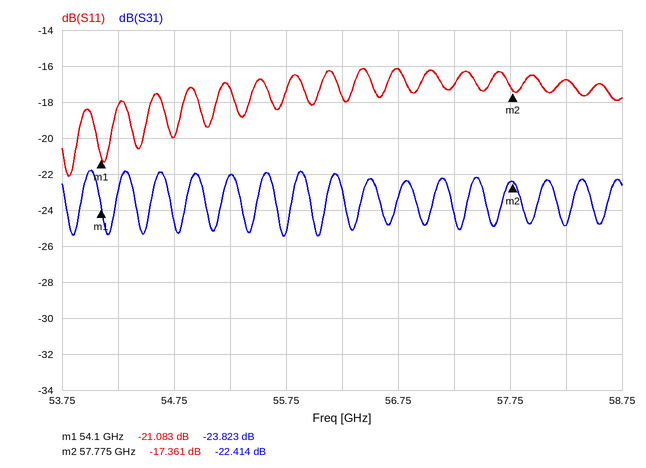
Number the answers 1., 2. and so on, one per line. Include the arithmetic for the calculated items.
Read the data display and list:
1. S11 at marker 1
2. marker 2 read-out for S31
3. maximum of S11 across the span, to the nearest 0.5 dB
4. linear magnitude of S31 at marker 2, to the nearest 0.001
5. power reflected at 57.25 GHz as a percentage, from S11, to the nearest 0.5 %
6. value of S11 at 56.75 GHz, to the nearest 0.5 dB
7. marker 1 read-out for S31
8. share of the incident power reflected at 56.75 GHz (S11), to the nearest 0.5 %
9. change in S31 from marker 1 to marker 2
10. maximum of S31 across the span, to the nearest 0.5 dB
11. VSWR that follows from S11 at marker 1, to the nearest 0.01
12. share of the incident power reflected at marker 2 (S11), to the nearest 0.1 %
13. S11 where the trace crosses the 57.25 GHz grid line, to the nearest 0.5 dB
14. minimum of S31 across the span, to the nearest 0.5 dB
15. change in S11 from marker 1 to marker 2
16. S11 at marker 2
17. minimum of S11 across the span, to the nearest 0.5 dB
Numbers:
1. -21.083 dB
2. -22.414 dB
3. -16.0 dB
4. 10^(-22.414/20) ≈ 0.076
5. 10^(-17/10) ≈ 2.0 %
6. -16.0 dB
7. -23.823 dB
8. 10^(-16/10) ≈ 2.5 %
9. -22.414 − (-23.823) = 1.409 dB
10. -22.0 dB
11. (1 + 0.0883)/(1 − 0.0883) ≈ 1.19
12. 10^(-17.361/10) ≈ 1.8 %
13. -17.0 dB
14. -25.5 dB
15. -17.361 − (-21.083) = 3.722 dB
16. -17.361 dB
17. -22.0 dB
